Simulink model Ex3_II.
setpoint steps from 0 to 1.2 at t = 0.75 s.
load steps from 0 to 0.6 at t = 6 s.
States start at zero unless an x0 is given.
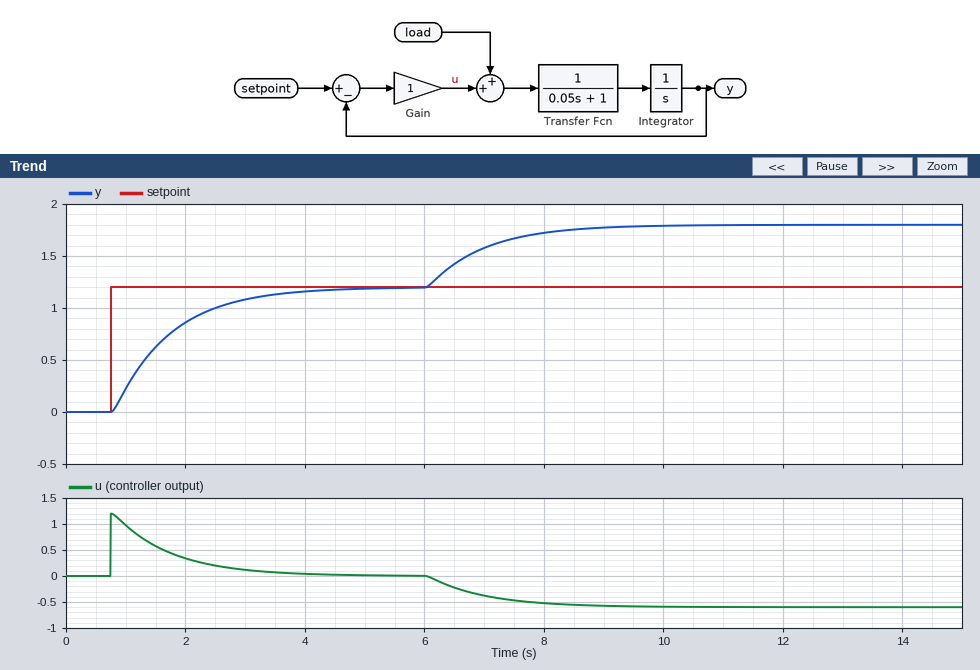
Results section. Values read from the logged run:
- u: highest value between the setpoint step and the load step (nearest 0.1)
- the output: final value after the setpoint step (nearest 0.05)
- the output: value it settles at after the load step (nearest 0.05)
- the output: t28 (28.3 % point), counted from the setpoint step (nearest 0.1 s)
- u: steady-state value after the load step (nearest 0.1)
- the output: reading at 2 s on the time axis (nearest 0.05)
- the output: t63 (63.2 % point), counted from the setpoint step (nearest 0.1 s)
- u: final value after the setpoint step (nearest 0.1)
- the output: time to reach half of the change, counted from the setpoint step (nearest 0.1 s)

1.2
1.20
1.80
0.4 s
-0.6
0.85
1.0 s
0.0
0.7 s
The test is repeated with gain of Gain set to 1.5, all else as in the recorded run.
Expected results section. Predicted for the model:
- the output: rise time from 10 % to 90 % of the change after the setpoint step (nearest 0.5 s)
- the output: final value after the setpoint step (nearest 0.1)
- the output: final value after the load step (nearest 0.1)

1.5 s
1.2
1.6
